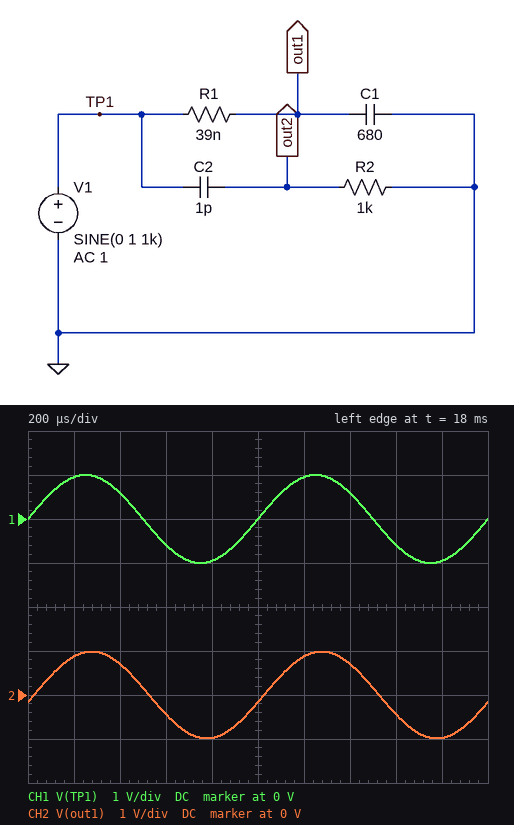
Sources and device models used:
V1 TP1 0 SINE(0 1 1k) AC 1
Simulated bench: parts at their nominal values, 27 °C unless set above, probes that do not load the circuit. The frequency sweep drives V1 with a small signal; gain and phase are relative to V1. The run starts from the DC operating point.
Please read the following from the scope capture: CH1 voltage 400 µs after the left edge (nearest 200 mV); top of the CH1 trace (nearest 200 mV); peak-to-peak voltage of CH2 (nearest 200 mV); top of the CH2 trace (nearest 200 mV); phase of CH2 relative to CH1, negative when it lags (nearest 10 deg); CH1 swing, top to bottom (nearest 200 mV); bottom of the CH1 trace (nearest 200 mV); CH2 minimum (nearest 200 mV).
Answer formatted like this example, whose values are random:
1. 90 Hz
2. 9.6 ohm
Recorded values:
1. 600 mV
2. 1.0 V
3. 2.0 V
4. 1.0 V
5. -10 deg
6. 2.0 V
7. -1.0 V
8. -1.0 V
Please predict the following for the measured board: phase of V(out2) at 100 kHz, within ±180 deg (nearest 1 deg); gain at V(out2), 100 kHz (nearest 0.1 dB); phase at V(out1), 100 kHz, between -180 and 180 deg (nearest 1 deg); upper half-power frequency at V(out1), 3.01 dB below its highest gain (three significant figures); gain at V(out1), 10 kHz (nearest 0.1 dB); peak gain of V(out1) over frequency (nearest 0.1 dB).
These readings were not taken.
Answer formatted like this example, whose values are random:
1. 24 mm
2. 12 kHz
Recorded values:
1. 90 deg
2. -64.0 dB
3. -87 deg
4. 6.00 kHz
5. -5.8 dB
6. 0 dB
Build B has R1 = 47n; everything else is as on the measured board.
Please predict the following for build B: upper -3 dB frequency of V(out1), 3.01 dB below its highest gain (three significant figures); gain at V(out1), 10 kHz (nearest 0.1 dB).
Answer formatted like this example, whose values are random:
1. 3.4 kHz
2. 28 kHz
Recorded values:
1. 4.98 kHz
2. -7.0 dB
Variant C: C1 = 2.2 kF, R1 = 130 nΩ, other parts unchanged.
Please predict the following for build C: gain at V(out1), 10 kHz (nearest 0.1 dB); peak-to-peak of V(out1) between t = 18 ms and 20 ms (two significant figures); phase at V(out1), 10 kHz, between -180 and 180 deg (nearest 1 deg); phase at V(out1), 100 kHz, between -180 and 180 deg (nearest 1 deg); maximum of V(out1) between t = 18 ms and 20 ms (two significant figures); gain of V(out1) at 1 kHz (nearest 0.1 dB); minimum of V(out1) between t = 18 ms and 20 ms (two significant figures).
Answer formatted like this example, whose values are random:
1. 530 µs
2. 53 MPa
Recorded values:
1. -25.1 dB
2. 970 mV
3. -87 deg
4. -90 deg
5. 490 mV
6. -6.3 dB
7. -490 mV
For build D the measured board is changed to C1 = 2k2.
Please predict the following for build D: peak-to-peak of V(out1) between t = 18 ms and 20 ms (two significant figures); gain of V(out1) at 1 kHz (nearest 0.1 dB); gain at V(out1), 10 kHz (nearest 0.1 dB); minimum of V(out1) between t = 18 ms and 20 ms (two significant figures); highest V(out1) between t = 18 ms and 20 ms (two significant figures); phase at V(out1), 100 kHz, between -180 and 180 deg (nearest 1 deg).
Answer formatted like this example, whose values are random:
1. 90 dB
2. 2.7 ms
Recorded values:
1. 1.8 V
2. -1.1 dB
3. -14.8 dB
4. -880 mV
5. 880 mV
6. -89 deg
